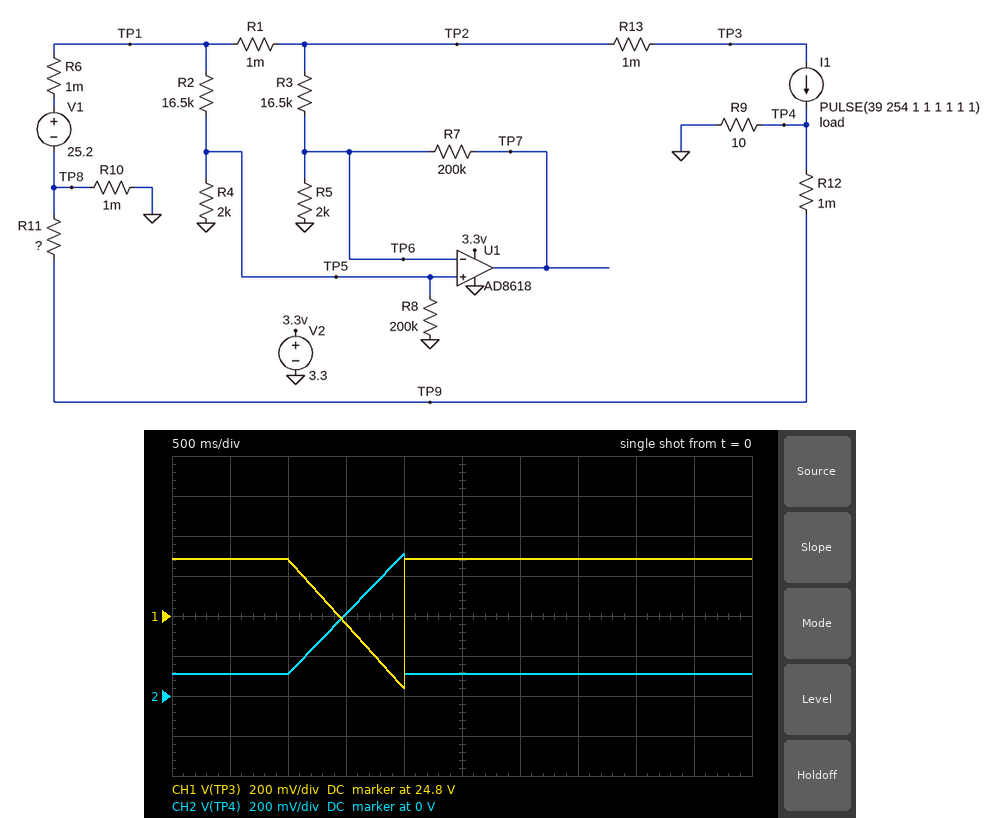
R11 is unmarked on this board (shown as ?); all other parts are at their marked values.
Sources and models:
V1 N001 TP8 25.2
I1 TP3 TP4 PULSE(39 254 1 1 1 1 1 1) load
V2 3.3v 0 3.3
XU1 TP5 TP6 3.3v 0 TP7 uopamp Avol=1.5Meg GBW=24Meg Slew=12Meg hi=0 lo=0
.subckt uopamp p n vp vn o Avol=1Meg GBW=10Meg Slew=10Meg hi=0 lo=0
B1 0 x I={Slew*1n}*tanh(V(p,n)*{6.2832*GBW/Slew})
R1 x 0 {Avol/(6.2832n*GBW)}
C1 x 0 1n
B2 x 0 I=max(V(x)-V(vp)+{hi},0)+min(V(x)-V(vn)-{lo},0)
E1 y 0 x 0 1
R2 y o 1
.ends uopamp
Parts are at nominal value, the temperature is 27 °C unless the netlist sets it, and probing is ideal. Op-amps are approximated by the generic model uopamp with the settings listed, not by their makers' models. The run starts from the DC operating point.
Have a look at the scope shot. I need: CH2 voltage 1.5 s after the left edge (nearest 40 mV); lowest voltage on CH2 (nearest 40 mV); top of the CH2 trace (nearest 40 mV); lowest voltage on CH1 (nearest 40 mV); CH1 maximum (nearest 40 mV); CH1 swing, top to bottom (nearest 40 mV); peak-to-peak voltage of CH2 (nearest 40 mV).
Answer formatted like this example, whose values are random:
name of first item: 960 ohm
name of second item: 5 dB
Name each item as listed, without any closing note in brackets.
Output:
CH2 voltage 1.5 s after the left edge: 400 mV
lowest voltage on CH2: 120 mV
top of the CH2 trace: 720 mV
lowest voltage on CH1: 24.44 V
CH1 maximum: 25.08 V
CH1 swing, top to bottom: 640 mV
peak-to-peak voltage of CH2: 600 mV
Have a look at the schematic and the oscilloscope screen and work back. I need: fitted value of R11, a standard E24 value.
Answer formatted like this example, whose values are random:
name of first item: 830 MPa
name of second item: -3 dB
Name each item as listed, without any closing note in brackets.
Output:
fitted value of R11, a standard E24 value: 1.8 mΩ
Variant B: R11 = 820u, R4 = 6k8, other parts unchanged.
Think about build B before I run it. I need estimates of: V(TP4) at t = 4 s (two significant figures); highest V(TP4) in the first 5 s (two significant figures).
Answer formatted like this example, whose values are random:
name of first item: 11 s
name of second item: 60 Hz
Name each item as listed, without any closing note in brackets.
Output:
V(TP4) at t = 4 s: 71 mV
highest V(TP4) in the first 5 s: 460 mV
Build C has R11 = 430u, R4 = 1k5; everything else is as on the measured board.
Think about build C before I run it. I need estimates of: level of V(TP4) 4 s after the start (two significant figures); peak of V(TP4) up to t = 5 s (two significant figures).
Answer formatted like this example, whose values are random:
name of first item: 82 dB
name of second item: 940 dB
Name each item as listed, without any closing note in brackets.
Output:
level of V(TP4) 4 s after the start: 56 mV
peak of V(TP4) up to t = 5 s: 360 mV
